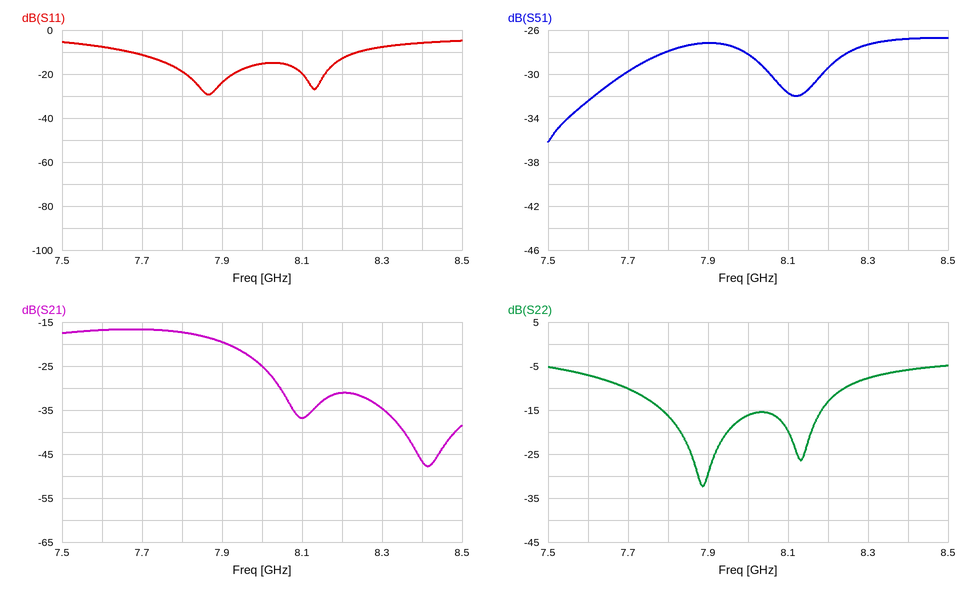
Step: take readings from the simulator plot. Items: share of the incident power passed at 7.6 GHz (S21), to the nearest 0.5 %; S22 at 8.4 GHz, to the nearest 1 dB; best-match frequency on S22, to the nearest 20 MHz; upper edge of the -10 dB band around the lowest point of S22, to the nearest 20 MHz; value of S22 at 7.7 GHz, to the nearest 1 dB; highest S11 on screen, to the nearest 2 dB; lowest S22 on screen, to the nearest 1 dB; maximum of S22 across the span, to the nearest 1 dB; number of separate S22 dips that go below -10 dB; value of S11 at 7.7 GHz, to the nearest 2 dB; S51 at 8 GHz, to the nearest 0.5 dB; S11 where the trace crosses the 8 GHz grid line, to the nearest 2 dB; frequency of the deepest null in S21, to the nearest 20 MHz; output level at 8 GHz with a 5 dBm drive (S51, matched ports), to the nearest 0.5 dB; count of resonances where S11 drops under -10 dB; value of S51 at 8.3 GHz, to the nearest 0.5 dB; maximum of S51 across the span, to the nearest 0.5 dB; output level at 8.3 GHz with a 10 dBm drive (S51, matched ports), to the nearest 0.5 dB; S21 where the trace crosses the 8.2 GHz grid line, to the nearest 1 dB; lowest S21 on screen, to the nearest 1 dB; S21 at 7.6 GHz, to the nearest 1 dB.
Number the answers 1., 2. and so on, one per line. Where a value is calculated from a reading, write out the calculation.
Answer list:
1. 10^(-17/10) ≈ 2.0 %
2. -6 dB
3. 7.88 GHz
4. 8.24 GHz
5. -10 dB
6. -4 dB
7. -32 dB
8. -5 dB
9. 2
10. -12 dB
11. -28.0 dB
12. -16 dB
13. 8.42 GHz
14. 5 dBm + (-28.0 dB) = -23.0 dBm
15. 2
16. -27.5 dB
17. -26.5 dB
18. 10 dBm + (-27.5 dB) = -17.5 dBm
19. -31 dB
20. -48 dB
21. -17 dB
